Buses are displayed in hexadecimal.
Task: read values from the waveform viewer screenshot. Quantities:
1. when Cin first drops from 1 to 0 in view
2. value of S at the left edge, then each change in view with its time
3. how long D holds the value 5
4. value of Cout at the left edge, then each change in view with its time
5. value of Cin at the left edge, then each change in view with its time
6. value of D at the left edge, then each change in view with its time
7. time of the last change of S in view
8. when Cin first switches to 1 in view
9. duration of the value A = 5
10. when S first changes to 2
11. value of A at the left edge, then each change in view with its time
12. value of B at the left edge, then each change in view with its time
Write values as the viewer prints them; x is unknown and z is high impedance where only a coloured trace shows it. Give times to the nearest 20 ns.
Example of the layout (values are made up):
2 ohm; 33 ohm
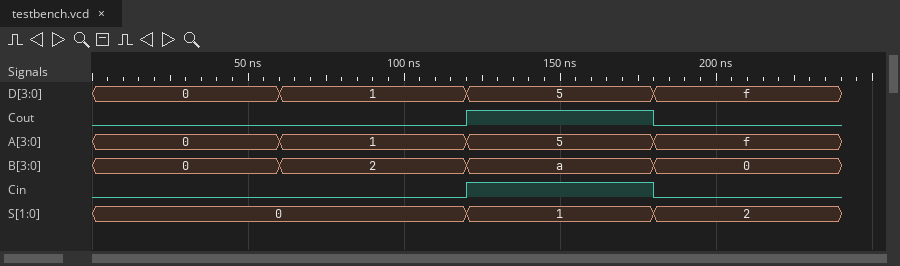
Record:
180 ns; 0, 1 at 120 ns, 2 at 180 ns; 60 ns; 0, 1 at 120 ns, 0 at 180 ns; 0, 1 at 120 ns, 0 at 180 ns; 0, 1 at 60 ns, 5 at 120 ns, f at 180 ns; 180 ns; 120 ns; 60 ns; 180 ns; 0, 1 at 60 ns, 5 at 120 ns, f at 180 ns; 0, 2 at 60 ns, a at 120 ns, 0 at 180 ns
